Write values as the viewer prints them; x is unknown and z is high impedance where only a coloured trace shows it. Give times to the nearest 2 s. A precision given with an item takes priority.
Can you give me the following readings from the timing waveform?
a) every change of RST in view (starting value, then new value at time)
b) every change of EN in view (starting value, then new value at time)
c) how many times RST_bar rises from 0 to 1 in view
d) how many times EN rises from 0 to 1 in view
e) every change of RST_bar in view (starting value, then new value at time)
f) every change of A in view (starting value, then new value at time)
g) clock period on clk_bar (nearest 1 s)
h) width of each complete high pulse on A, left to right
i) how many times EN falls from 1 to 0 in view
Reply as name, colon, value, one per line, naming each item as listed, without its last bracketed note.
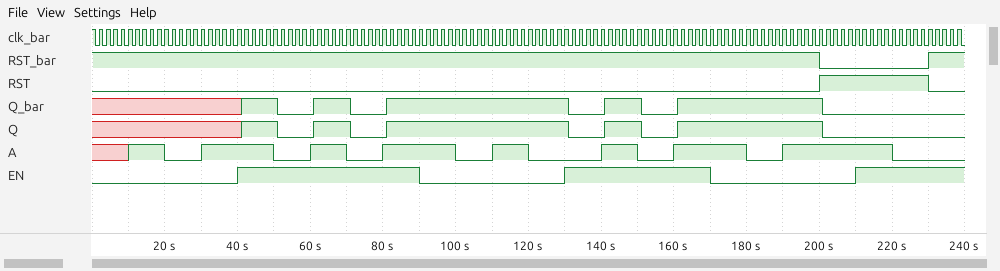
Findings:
every change of RST in view: 0, 1 at 200 s, 0 at 230 s
every change of EN in view: 0, 1 at 40 s, 0 at 90 s, 1 at 130 s, 0 at 170 s, 1 at 210 s
how many times RST_bar rises from 0 to 1 in view: 1
how many times EN rises from 0 to 1 in view: 3
every change of RST_bar in view: 1, 0 at 200 s, 1 at 230 s
every change of A in view: x, 1 at 10 s, 0 at 20 s, 1 at 30 s, 0 at 50 s, 1 at 60 s, 0 at 70 s, 1 at 80 s, 0 at 100 s, 1 at 110 s, 0 at 120 s, 1 at 140 s, 0 at 150 s, 1 at 160 s, 0 at 180 s, 1 at 190 s, 0 at 220 s
clock period on clk_bar: 2 s
width of each complete high pulse on A, left to right: 20 s, 10 s, 20 s, 10 s, 10 s, 20 s, 30 s
how many times EN falls from 1 to 0 in view: 2
